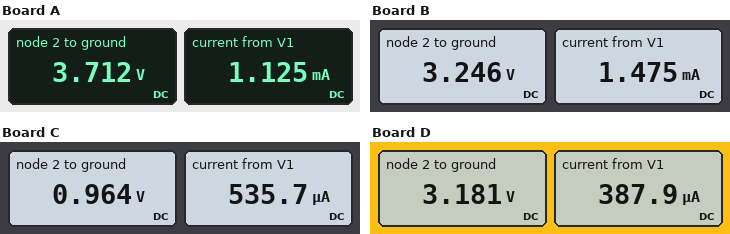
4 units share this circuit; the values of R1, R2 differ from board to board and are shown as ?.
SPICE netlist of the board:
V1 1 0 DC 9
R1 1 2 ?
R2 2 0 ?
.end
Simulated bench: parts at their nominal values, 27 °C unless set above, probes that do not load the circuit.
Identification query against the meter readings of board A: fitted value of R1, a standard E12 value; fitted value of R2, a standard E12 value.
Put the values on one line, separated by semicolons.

4.7 kΩ; 3.3 kΩ
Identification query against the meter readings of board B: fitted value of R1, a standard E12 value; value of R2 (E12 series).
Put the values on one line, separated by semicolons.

3.9 kΩ; 2.2 kΩ
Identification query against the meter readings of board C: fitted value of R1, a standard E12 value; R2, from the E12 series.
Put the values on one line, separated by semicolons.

15 kΩ; 1.8 kΩ
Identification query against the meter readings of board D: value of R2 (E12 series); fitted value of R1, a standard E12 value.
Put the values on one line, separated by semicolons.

8.2 kΩ; 15 kΩ
